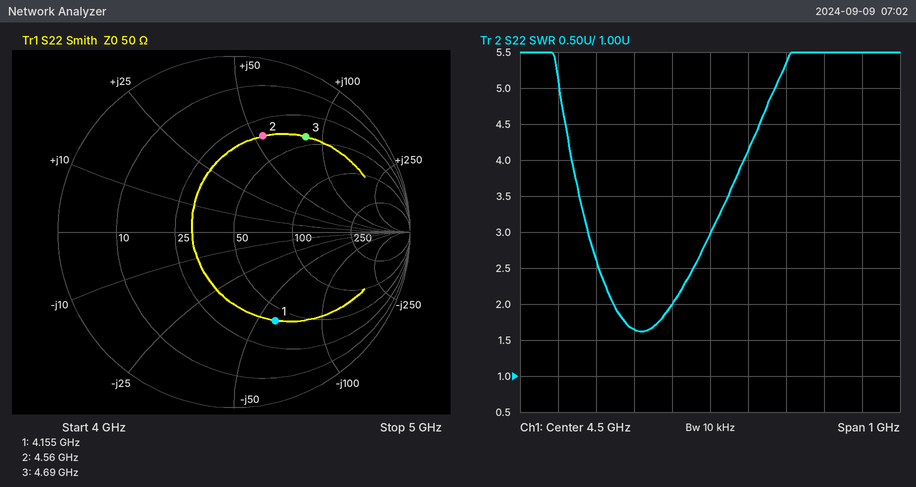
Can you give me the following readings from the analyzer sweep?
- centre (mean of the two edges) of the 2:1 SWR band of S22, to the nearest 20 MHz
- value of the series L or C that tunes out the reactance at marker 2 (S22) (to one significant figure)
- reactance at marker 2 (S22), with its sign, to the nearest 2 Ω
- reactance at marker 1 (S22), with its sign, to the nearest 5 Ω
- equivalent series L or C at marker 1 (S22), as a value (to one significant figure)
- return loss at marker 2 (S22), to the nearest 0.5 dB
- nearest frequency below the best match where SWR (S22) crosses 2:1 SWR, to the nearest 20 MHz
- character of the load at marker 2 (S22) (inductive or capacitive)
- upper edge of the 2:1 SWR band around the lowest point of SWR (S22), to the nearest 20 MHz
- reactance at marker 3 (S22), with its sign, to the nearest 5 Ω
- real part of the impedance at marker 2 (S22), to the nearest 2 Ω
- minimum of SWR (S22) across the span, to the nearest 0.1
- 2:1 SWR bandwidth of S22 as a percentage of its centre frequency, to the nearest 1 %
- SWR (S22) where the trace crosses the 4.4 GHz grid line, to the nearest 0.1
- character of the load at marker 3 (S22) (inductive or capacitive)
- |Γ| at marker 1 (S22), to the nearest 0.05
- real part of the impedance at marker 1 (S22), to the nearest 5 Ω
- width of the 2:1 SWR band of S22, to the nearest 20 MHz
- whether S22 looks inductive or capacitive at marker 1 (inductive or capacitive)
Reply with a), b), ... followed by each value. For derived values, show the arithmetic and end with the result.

a) 4.32 GHz
b) C = 1/(2π × 4.56 GHz × 54 Ω) ≈ 646 fF, so 600 fF to one significant figure
c) +54 Ω
d) -60 Ω
e) C = 1/(2π × 4.155 GHz × 60 Ω) ≈ 638 fF, so 600 fF to one significant figure
f) 5.0 dB
g) 4.24 GHz
h) inductive
i) 4.40 GHz
j) +85 Ω
k) 34 Ω
l) 1.6
m) 160 MHz / 4.32 GHz ≈ 4 %
n) 2.0
o) inductive
p) 0.55
q) 40 Ω
r) 4.40 GHz − 4.24 GHz = 160 MHz
s) capacitive
